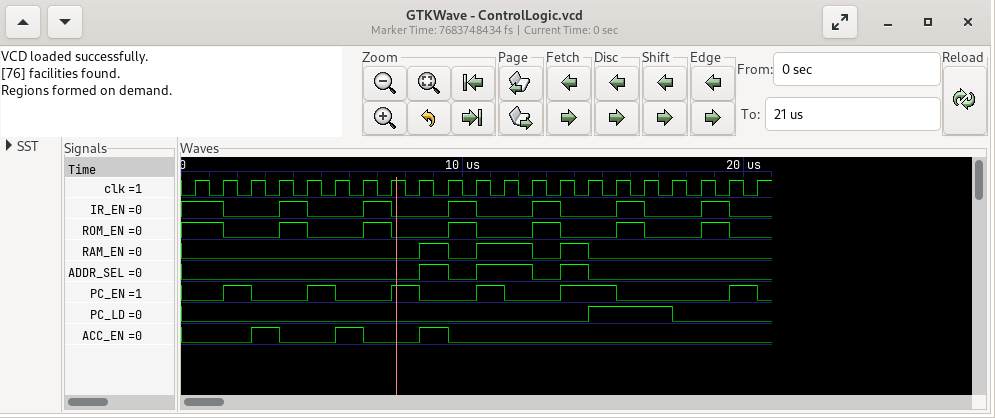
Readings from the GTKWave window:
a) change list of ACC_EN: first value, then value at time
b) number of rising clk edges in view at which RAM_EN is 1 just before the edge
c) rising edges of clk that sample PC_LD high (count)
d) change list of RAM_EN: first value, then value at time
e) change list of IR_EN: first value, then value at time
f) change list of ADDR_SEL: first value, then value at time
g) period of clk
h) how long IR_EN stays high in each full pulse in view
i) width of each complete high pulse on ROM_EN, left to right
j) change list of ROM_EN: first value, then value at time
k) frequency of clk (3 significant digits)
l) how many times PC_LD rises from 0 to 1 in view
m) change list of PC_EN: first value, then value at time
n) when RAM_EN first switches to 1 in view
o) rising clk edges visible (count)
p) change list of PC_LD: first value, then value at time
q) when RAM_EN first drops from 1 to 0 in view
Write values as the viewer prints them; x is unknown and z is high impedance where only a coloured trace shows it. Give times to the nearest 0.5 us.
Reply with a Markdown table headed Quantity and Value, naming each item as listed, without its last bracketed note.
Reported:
| Quantity | Value |
|---|---|
| change list of ACC_EN: first value, then value at time | 0, 1 at 2.5 us, 0 at 3.5 us, 1 at 5.5 us, 0 at 6.5 us, 1 at 8.5 us, 0 at 9.5 us |
| number of rising clk edges in view at which RAM_EN is 1 just before the edge | 4 |
| rising edges of clk that sample PC_LD high | 3 |
| change list of RAM_EN: first value, then value at time | 0, 1 at 8.5 us, 0 at 9.5 us, 1 at 10.5 us, 0 at 12.5 us, 1 at 13.5 us, 0 at 14.5 us |
| change list of IR_EN: first value, then value at time | 1, 0 at 1.5 us, 1 at 3.5 us, 0 at 4.5 us, 1 at 6.5 us, 0 at 7.5 us, 1 at 9.5 us, 0 at 10.5 us, 1 at 12.5 us, 0 at 13.5 us, 1 at 15.5 us, 0 at 16.5 us, 1 at 18.5 us, 0 at 19.5 us |
| change list of ADDR_SEL: first value, then value at time | 0, 1 at 8.5 us, 0 at 9.5 us, 1 at 10.5 us, 0 at 12.5 us, 1 at 13.5 us, 0 at 14.5 us |
| period of clk | 1 us |
| how long IR_EN stays high in each full pulse in view | 1 us, 1 us, 1 us, 1 us, 1 us, 1 us |
| width of each complete high pulse on ROM_EN, left to right | 1 us, 1 us, 1 us, 1 us, 1 us, 1 us |
| change list of ROM_EN: first value, then value at time | 1, 0 at 1.5 us, 1 at 3.5 us, 0 at 4.5 us, 1 at 6.5 us, 0 at 7.5 us, 1 at 9.5 us, 0 at 10.5 us, 1 at 12.5 us, 0 at 13.5 us, 1 at 15.5 us, 0 at 16.5 us, 1 at 18.5 us, 0 at 19.5 us |
| frequency of clk | 1.00 MHz |
| how many times PC_LD rises from 0 to 1 in view | 1 |
| change list of PC_EN: first value, then value at time | 0, 1 at 1.5 us, 0 at 2.5 us, 1 at 4.5 us, 0 at 5.5 us, 1 at 7.5 us, 0 at 8.5 us, 1 at 10.5 us, 0 at 11.5 us, 1 at 13.5 us, 0 at 15.5 us, 1 at 19.5 us, 0 at 20.5 us |
| when RAM_EN first switches to 1 in view | 8.5 us |
| rising clk edges visible | 21 |
| change list of PC_LD: first value, then value at time | 0, 1 at 14.5 us, 0 at 17.5 us |
| when RAM_EN first drops from 1 to 0 in view | 9.5 us |
